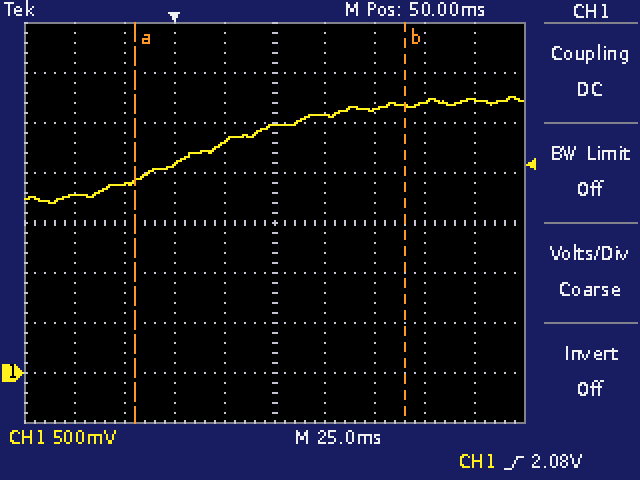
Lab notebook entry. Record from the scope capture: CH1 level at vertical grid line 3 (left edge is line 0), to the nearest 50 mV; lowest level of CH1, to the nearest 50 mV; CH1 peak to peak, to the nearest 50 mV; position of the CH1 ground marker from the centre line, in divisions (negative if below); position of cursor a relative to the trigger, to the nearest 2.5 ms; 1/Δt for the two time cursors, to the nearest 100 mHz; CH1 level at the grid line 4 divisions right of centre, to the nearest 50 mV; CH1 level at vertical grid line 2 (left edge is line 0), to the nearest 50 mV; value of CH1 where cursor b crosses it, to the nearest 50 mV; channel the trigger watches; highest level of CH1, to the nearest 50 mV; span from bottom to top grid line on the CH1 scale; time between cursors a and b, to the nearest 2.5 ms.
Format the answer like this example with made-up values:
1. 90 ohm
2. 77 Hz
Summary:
1. 2.10 V
2. 1.70 V
3. 1.05 V
4. -3.0 div
5. -20.0 ms
6. 7.4 Hz
7. 2.75 V
8. 1.90 V
9. 2.65 V
10. CH1
11. 2.75 V
12. 4 V
13. 135.0 ms
